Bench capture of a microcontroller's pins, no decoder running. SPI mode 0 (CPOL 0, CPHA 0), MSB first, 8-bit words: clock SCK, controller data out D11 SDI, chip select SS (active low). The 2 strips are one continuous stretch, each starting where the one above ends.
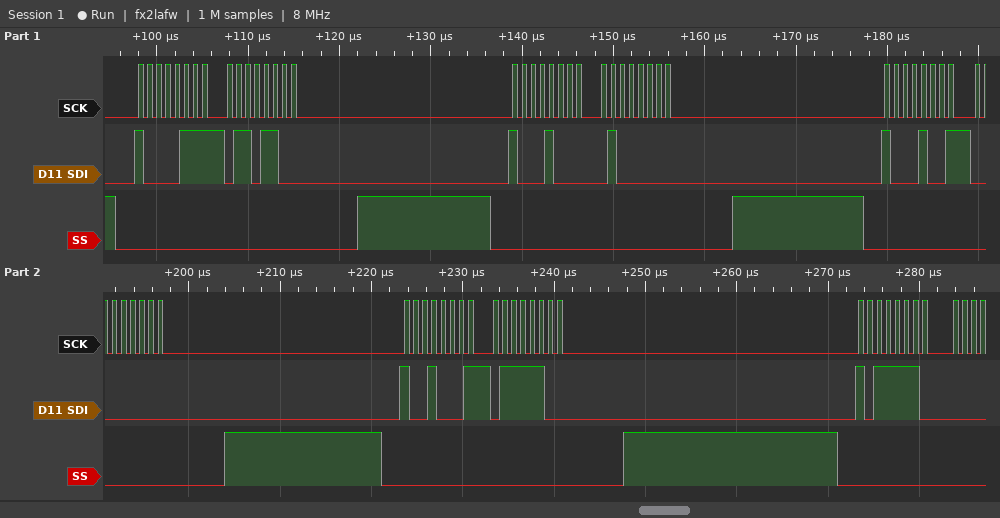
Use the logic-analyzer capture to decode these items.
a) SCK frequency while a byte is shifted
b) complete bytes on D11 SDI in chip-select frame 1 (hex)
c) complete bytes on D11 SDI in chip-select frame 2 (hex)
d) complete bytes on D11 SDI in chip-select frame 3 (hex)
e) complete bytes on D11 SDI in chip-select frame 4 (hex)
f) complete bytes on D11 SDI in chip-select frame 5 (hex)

1 MHz
87 6C
88 40
89 00
91 7C
BE
